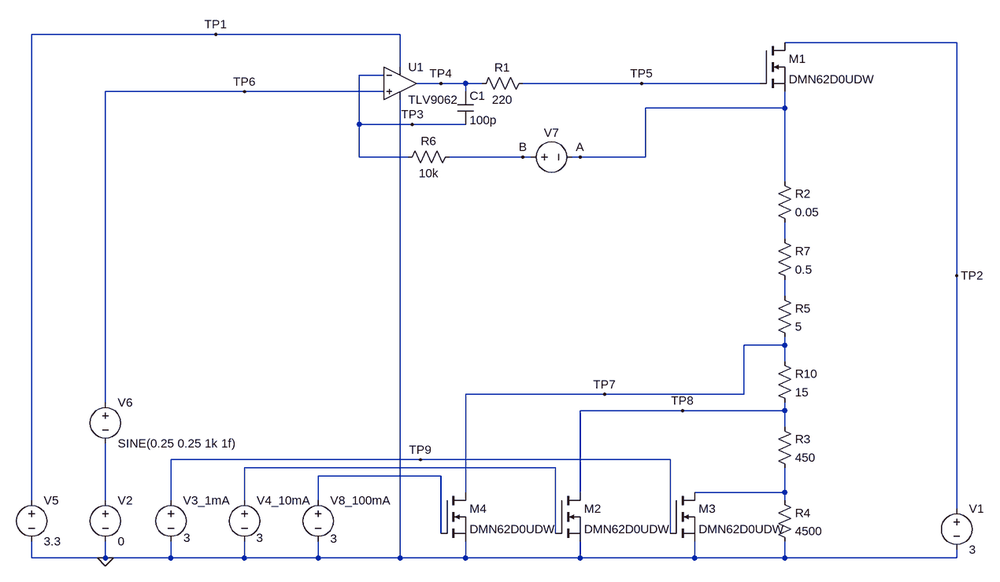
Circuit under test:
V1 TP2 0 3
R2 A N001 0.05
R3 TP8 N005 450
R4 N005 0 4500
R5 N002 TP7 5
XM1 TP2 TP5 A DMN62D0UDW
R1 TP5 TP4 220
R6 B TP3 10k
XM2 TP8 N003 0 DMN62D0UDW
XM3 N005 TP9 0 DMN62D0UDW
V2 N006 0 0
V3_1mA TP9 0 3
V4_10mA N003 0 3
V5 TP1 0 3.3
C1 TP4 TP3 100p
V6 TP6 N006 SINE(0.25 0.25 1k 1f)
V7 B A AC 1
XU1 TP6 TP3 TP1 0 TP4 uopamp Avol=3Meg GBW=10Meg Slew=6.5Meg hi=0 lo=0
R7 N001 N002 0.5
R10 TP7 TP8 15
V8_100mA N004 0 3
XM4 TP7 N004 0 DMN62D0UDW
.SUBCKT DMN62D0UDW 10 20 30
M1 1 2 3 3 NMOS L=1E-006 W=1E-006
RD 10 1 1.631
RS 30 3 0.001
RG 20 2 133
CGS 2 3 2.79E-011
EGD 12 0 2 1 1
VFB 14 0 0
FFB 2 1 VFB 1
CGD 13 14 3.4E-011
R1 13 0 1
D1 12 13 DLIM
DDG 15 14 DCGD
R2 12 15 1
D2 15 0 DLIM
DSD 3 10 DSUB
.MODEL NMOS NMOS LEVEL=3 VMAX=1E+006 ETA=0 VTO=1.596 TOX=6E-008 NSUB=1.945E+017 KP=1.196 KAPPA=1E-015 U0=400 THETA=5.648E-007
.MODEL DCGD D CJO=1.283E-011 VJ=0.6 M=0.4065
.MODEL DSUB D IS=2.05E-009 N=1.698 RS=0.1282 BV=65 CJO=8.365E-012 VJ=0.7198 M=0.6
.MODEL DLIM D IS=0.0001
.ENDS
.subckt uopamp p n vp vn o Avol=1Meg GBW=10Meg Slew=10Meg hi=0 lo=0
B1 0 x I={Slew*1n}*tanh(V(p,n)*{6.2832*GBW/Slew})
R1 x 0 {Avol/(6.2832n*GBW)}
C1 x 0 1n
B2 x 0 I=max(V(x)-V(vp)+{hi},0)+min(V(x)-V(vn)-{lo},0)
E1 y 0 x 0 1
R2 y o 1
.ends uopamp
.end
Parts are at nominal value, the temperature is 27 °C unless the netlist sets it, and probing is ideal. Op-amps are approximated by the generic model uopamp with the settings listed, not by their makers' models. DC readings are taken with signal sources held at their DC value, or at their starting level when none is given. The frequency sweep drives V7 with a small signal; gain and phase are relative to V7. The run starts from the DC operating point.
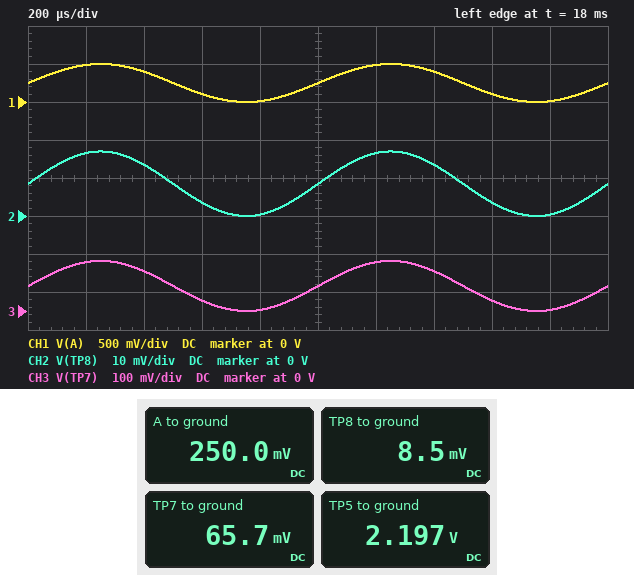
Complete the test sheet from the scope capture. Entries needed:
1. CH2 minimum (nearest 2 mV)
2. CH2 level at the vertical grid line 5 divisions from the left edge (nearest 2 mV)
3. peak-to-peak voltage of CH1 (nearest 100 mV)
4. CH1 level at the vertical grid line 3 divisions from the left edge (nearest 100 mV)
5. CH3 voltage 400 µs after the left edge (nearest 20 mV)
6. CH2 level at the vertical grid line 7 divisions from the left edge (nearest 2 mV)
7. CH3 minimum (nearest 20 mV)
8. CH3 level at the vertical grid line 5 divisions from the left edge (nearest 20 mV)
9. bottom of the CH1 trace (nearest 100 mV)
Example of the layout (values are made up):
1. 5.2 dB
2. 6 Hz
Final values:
1. 0 V
2. 8 mV
3. 500 mV
4. 100 mV
5. 100 mV
6. 14 mV
7. 0 V
8. 60 mV
9. 0 V
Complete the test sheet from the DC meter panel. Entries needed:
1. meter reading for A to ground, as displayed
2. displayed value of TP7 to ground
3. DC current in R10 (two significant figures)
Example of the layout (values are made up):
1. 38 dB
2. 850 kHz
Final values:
1. 250.0 mV
2. 65.7 mV
3. 3.8 mA
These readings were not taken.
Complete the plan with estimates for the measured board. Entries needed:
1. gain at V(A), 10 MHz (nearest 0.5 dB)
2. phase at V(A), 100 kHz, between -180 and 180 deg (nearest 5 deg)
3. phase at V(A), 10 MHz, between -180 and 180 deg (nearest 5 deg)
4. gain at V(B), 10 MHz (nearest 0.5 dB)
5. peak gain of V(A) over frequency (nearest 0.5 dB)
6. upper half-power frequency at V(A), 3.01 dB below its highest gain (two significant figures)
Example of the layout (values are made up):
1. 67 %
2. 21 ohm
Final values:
1. -45.0 dB
2. 130 deg
3. 20 deg
4. 0 dB
5. 0 dB
6. 93 kHz
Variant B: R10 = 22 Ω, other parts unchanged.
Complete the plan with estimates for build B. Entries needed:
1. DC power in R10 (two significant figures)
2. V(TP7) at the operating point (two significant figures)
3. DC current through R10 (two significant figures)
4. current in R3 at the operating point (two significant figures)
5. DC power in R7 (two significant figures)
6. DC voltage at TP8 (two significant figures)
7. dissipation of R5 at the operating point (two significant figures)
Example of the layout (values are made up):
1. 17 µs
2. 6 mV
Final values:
1. 170 µW
2. 67 mV
3. 2.8 mA
4. 14 µA
5. 540 µW
6. 6.2 mV
7. 5.4 mW
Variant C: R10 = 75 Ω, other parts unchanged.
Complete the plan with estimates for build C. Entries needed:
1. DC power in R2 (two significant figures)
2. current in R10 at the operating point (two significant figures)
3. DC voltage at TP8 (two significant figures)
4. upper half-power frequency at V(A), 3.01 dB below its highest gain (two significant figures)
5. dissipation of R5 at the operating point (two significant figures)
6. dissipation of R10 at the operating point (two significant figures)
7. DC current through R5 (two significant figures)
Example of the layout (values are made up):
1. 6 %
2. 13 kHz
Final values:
1. 52 µW
2. 910 µA
3. 2.0 mV
4. 94 kHz
5. 5.2 mW
6. 62 µW
7. 32 mA
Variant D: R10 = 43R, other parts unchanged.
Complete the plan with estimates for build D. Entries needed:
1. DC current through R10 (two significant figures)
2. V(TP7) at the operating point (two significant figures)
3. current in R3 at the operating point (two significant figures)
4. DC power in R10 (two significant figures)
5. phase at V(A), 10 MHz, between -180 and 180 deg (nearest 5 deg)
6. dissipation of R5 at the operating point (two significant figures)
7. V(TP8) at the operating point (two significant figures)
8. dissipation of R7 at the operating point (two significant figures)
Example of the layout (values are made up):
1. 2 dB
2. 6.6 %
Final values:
1. 1.5 mA
2. 69 mV
3. 7.5 µA
4. 100 µW
5. 20 deg
6. 5.3 mW
7. 3.4 mV
8. 530 µW
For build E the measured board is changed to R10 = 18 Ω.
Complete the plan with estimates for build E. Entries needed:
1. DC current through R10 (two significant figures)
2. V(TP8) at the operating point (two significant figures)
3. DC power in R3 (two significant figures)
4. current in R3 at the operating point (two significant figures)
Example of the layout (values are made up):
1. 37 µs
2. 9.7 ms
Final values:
1. 3.3 mA
2. 7.3 mV
3. 120 nW
4. 16 µA
